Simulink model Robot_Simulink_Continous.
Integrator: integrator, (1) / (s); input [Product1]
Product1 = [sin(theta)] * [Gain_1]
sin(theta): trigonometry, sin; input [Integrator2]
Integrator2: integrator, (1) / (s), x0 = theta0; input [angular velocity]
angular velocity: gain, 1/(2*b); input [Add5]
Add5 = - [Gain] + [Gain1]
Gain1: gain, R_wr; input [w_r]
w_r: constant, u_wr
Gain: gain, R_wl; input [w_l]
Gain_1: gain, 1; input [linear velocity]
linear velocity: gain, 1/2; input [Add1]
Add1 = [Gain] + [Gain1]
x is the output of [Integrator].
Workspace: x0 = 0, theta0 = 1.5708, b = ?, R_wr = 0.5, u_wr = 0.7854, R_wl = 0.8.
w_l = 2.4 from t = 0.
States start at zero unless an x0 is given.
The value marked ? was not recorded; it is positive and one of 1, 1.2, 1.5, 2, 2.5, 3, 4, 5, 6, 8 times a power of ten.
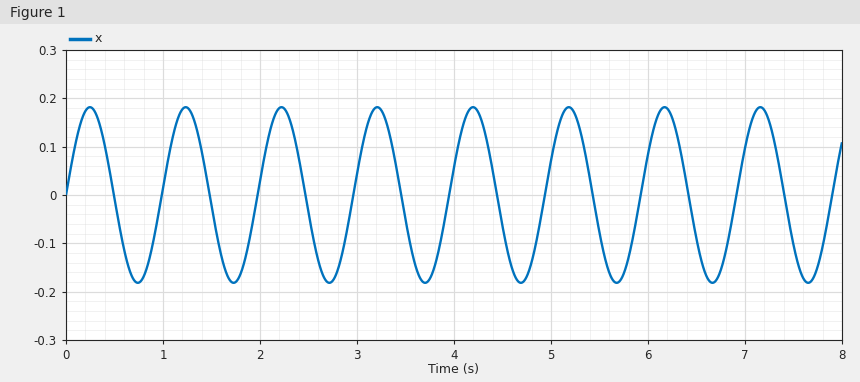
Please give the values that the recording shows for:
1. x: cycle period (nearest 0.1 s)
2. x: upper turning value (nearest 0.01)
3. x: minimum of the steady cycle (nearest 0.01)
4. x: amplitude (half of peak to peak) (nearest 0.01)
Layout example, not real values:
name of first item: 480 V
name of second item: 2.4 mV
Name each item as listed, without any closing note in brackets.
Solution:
x: cycle period: 1.0 s
x: upper turning value: 0.18
x: minimum of the steady cycle: -0.18
x: amplitude (half of peak to peak): 0.18
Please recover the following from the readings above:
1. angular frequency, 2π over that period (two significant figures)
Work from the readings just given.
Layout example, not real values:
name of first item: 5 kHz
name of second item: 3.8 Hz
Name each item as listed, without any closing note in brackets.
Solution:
angular frequency, 2π over that period: 6.3 rad/s
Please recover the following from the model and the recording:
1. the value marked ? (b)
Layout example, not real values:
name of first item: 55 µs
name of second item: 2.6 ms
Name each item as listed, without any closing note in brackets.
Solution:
the value marked ?: 0.12
